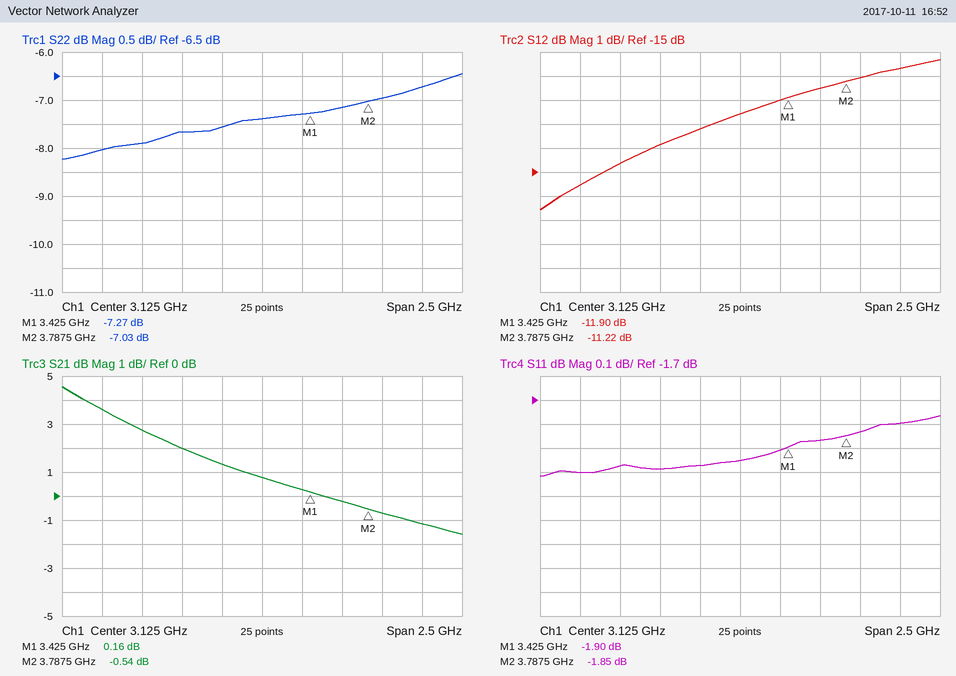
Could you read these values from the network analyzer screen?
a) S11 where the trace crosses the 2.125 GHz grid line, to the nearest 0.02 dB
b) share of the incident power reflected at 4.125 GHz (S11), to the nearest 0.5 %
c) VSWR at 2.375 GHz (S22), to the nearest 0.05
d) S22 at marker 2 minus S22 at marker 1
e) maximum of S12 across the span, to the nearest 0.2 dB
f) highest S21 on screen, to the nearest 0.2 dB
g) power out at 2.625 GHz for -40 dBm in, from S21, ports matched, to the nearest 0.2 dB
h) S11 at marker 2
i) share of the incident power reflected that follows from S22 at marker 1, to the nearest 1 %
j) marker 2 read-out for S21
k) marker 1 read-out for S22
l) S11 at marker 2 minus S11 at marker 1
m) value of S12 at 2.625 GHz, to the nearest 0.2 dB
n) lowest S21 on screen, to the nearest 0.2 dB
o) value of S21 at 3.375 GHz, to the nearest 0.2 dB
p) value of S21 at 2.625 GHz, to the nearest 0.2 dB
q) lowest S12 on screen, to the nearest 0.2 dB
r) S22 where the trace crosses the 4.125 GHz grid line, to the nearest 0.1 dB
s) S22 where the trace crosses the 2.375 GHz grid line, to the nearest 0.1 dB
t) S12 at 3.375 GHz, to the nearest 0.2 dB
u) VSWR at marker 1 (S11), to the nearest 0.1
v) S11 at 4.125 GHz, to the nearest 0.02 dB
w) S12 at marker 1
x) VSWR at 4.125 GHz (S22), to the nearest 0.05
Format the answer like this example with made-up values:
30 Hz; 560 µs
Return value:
-2.00 dB; 66.0 %; 2.35; 0.24 dB; -10.4 dB; 4.6 dB; -38.0 dBm; -1.85 dB; 19 %; -0.54 dB; -7.27 dB; 0.05 dB; -13.8 dB; -1.6 dB; 0.2 dB; 2.0 dB; -16.6 dB; -6.7 dB; -7.9 dB; -12.0 dB; 9.2; -1.80 dB; -11.90 dB; 2.70
